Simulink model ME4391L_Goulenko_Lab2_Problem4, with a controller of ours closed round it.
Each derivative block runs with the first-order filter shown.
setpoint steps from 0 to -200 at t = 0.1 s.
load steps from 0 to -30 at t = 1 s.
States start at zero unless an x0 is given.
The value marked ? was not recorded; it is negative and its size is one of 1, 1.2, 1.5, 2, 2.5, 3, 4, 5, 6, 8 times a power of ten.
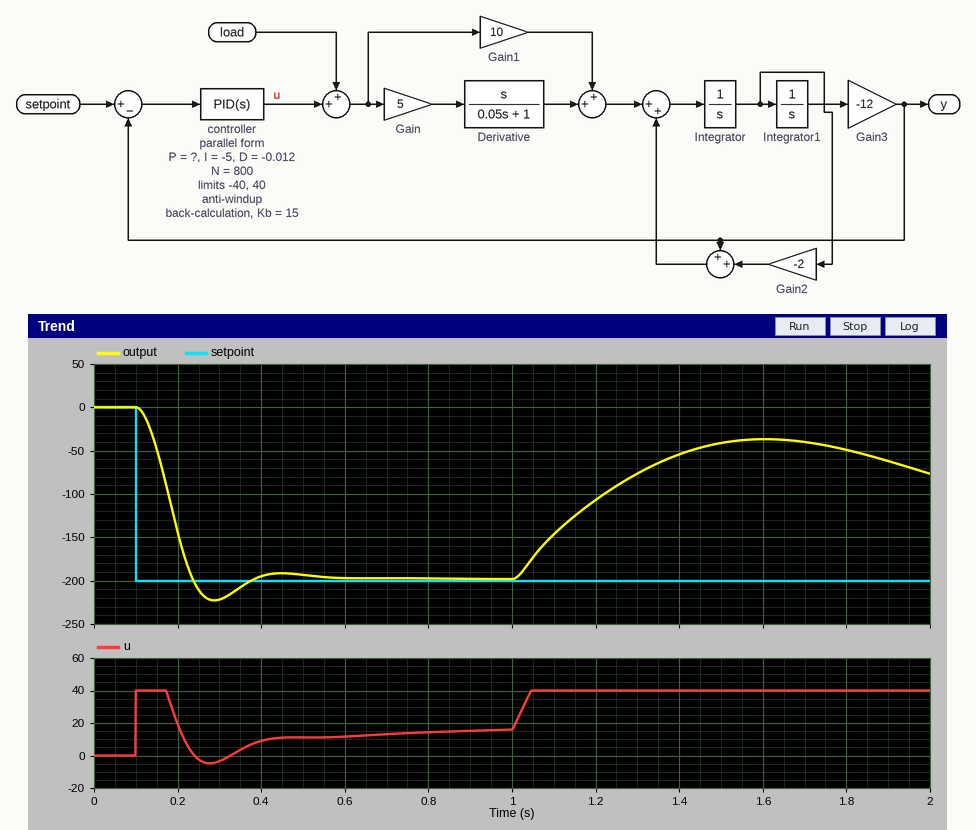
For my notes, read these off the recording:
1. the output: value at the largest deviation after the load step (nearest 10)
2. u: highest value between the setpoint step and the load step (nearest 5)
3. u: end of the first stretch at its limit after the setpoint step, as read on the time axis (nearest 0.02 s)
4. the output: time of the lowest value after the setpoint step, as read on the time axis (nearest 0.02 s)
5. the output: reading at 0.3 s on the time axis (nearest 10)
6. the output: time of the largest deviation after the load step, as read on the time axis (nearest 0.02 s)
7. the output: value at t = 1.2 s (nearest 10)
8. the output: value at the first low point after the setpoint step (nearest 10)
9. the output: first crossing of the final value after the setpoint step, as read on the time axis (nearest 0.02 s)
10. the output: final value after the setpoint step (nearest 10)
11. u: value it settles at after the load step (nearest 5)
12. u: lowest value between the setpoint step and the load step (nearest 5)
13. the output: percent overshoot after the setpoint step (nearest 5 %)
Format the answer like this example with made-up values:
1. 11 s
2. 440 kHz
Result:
1. -40
2. 40
3. 0.18 s
4. 0.28 s
5. -220
6. 1.60 s
7. -110
8. -220
9. 0.24 s
10. -200
11. 40
12. -5
13. 10 %
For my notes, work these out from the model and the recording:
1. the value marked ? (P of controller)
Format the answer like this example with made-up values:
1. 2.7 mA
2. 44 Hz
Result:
1. -0.6
